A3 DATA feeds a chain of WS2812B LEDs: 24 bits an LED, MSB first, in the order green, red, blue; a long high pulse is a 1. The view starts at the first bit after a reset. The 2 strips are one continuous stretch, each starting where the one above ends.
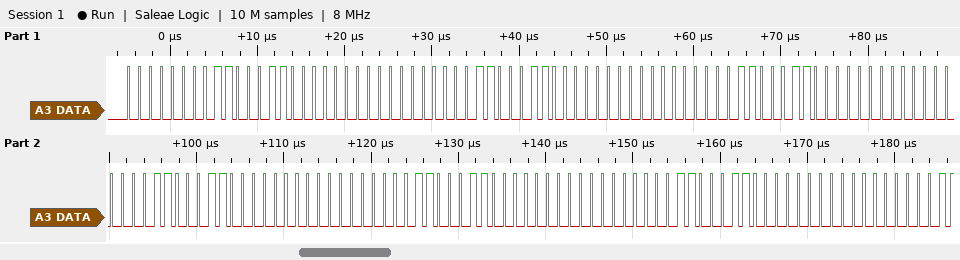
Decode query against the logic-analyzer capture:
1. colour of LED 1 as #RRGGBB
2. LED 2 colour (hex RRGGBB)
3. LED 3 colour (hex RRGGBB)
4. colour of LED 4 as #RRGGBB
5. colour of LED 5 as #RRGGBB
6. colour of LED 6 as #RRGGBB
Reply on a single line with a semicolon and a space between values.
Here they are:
#C60000; #C60000; #C60000; #C60000; #C60000; #C60000
